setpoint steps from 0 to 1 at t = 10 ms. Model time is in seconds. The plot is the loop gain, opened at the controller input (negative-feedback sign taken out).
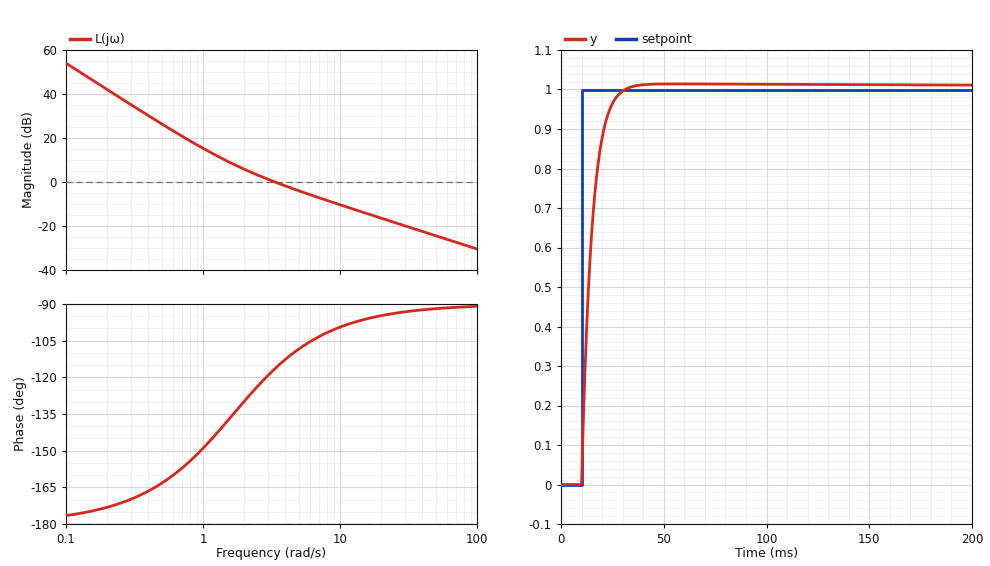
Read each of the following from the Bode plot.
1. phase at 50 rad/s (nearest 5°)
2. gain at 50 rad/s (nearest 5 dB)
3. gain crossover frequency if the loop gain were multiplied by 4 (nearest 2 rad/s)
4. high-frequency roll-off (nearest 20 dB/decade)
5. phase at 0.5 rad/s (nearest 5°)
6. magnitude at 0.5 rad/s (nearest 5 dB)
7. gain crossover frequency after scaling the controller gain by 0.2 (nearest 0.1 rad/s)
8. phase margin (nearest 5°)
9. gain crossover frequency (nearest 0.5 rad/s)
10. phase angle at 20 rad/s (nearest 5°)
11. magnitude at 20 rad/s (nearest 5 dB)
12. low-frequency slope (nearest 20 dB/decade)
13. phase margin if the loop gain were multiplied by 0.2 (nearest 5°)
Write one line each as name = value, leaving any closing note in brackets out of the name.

phase at 50 rad/s = -90°
gain at 50 rad/s = -25 dB
gain crossover frequency if the loop gain were multiplied by 4 = 12 rad/s
high-frequency roll-off = -20 dB/decade
phase at 0.5 rad/s = -165°
magnitude at 0.5 rad/s = 25 dB
gain crossover frequency after scaling the controller gain by 0.2 = 1.1 rad/s
phase margin = 65°
gain crossover frequency = 3.5 rad/s
phase angle at 20 rad/s = -95°
magnitude at 20 rad/s = -15 dB
low-frequency slope = -40 dB/decade
phase margin if the loop gain were multiplied by 0.2 = 35°
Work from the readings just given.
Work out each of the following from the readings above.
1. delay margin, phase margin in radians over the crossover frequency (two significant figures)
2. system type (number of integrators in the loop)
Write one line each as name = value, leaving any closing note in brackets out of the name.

delay margin, phase margin in radians over the crossover frequency = 0.32 s
system type = 2
